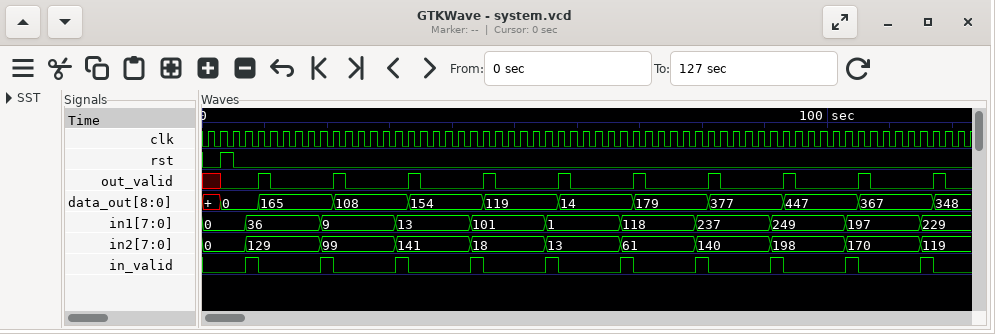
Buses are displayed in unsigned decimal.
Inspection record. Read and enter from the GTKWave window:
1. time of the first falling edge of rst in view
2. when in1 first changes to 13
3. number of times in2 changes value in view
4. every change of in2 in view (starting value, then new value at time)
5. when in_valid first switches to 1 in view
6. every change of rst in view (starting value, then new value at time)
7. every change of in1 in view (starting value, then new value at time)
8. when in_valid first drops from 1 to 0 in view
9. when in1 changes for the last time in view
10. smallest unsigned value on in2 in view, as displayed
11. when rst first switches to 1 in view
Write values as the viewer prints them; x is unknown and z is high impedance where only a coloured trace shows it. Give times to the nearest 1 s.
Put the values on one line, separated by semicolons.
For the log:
5 s; 31 s; 10; 0, 129 at 7 s, 99 at 19 s, 141 at 31 s, 18 at 43 s, 13 at 55 s, 61 at 67 s, 140 at 79 s, 198 at 91 s, 170 at 103 s, 119 at 115 s; 7 s; 0, 1 at 3 s, 0 at 5 s; 0, 36 at 7 s, 9 at 19 s, 13 at 31 s, 101 at 43 s, 1 at 55 s, 118 at 67 s, 237 at 79 s, 249 at 91 s, 197 at 103 s, 229 at 115 s; 9 s; 115 s; 0; 3 s
